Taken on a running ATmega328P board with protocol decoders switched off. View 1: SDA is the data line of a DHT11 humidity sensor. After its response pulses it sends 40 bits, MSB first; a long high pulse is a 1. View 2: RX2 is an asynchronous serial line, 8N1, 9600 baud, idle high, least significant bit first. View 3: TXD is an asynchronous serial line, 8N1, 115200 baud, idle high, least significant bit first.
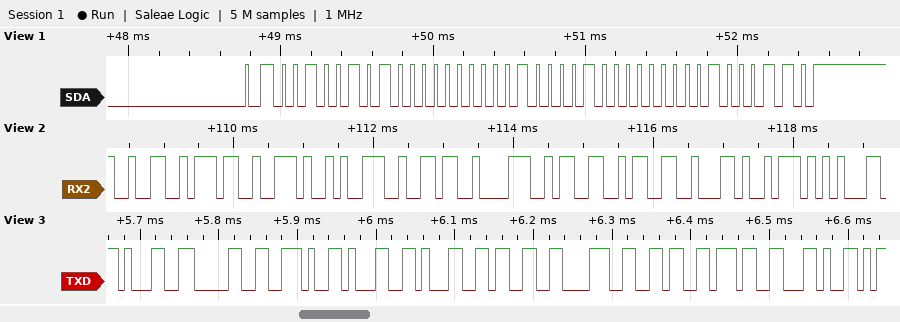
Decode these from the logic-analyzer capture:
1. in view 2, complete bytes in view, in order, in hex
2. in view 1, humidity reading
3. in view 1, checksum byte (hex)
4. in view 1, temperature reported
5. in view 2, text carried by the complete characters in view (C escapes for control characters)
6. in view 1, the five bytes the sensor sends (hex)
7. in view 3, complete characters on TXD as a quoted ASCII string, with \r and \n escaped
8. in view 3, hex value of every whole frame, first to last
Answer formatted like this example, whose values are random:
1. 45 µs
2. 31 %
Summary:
1. 32 37 2E 39 36 38 33 33 2C 57
2. 37 %
3. 0x46
4. 33.0 °C
5. "27.96833,W"
6. 25 00 21 00 46
7. "10.113867,"
8. 31 30 2E 31 31 33 38 36 37 2C
